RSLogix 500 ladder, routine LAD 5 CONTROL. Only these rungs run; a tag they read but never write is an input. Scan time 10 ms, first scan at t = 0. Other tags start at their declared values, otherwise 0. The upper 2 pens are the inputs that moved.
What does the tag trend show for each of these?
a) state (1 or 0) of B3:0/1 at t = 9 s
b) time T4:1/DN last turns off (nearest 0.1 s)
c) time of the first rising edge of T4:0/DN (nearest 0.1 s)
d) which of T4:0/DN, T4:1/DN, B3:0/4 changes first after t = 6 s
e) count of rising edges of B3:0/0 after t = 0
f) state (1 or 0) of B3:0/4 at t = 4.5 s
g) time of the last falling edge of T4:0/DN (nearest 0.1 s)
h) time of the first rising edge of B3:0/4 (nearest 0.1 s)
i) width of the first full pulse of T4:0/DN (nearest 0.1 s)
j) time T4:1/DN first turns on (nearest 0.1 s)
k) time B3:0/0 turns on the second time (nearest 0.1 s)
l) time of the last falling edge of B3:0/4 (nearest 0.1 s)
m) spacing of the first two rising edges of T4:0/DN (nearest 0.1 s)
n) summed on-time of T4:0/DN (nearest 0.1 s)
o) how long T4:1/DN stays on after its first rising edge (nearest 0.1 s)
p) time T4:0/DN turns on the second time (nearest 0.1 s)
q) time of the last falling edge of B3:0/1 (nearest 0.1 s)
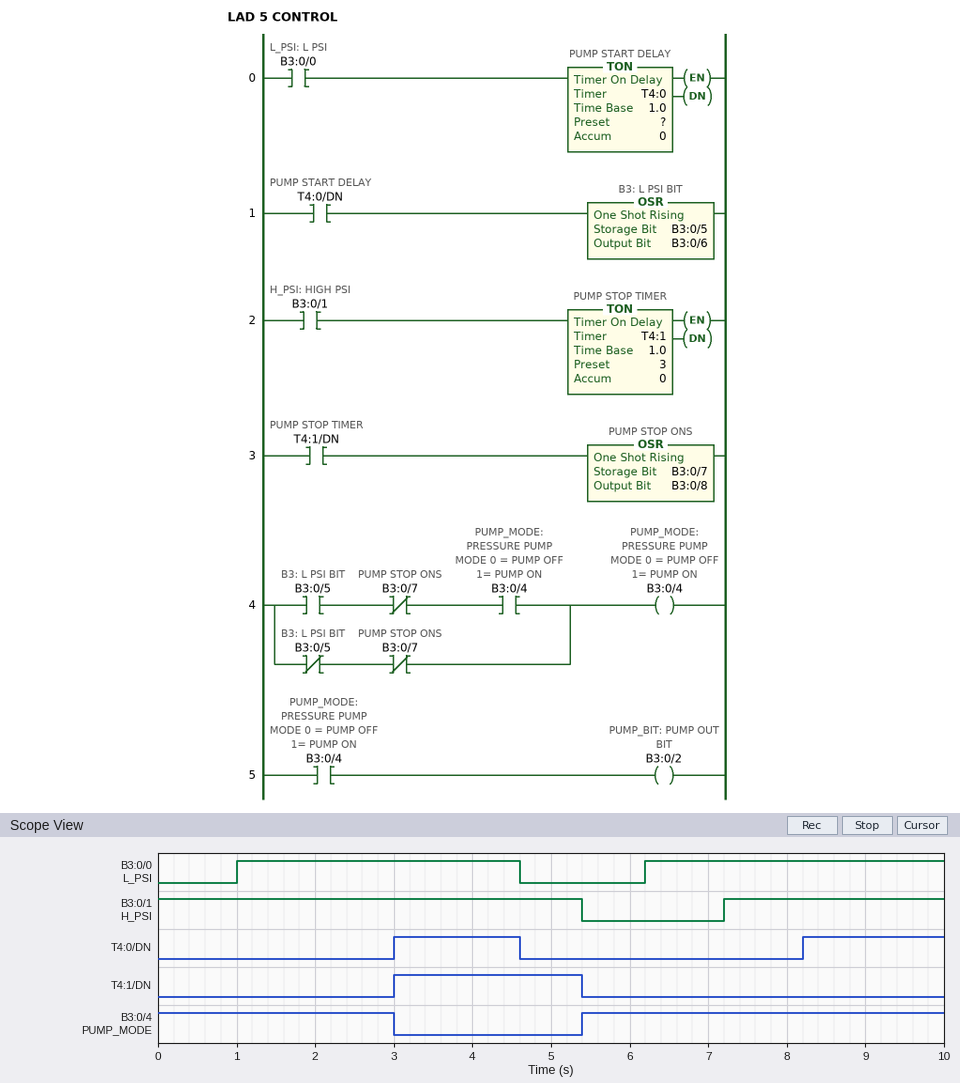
1
5.4 s
3.0 s
T4:0/DN
2
0
4.6 s
5.4 s
1.6 s
3.0 s
6.2 s
3.0 s
5.2 s
3.4 s
2.4 s
8.2 s
5.4 s
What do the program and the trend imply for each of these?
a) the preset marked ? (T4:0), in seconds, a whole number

2 s
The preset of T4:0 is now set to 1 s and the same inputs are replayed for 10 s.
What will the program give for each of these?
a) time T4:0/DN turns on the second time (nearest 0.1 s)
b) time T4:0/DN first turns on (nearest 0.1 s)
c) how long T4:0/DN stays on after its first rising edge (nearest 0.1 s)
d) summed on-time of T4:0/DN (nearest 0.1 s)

7.2 s
2.0 s
2.6 s
5.4 s
